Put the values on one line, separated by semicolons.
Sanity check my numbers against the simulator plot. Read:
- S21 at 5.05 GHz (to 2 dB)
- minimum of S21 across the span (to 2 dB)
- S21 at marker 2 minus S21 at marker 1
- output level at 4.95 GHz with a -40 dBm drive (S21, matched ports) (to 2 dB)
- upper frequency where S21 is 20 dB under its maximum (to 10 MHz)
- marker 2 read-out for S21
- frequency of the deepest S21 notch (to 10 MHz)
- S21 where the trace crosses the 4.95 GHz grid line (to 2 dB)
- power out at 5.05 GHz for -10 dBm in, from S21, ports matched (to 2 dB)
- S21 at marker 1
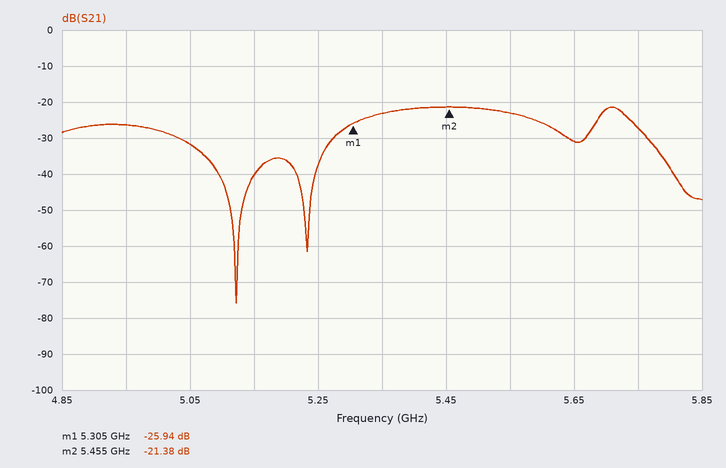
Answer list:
-32 dB; -76 dB; 4.56 dB; -66 dBm; 5.81 GHz; -21.38 dB; 5.12 GHz; -26 dB; -42 dBm; -25.94 dB
